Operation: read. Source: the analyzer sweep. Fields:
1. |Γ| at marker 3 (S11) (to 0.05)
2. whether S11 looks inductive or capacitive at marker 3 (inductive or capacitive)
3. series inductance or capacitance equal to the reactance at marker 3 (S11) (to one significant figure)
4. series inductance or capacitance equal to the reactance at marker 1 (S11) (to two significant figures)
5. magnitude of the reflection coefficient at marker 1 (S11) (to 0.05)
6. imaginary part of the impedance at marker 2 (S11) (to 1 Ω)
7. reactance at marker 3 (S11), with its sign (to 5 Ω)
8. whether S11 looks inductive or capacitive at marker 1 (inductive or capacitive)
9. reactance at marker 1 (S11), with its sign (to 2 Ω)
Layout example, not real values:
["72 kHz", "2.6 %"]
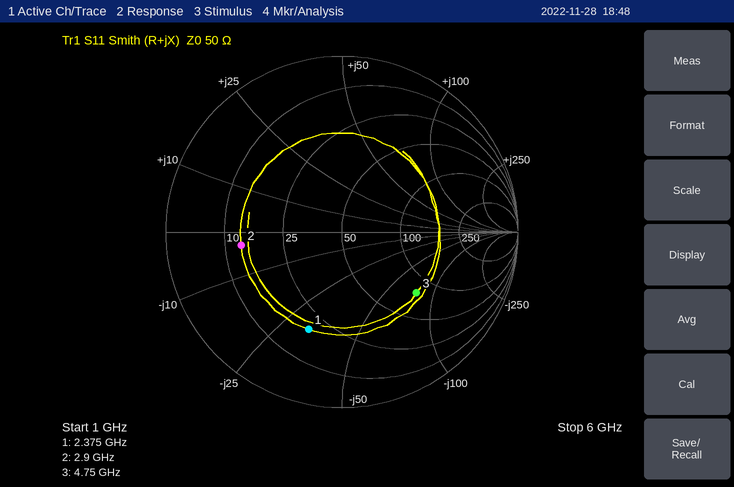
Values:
["0.55", "capacitive", "400 fF", "2.1 pF", "0.60", "-3 Ω", "-75 Ω", "capacitive", "-32 Ω"]
